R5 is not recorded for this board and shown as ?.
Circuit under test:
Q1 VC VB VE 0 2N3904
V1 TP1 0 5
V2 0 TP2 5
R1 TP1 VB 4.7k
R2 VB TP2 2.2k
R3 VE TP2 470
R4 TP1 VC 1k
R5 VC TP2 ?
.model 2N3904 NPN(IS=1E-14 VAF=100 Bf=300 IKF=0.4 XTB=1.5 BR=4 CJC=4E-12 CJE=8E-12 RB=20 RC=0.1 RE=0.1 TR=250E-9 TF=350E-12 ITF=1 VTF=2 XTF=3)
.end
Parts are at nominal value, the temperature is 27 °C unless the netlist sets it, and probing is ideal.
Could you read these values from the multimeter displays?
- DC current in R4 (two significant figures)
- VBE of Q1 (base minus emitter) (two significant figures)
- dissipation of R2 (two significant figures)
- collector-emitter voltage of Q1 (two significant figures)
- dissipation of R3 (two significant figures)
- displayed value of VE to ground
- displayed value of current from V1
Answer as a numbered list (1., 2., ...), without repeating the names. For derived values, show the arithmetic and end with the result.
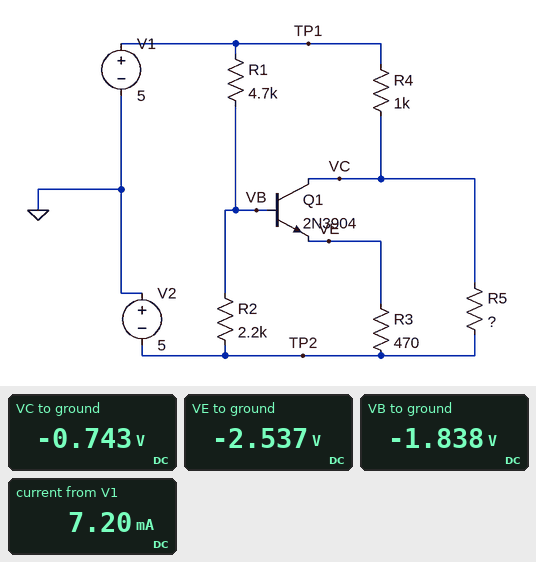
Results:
1. (5 V - (-743 mV)) / 1 kΩ = 5.7 mA
2. -1.838 V - (-2.537 V) = 700 mV
3. (-1.838 V - (-5 V))^2 / 2.2 kΩ = 4.5 mW
4. -743 mV - (-2.537 V) = 1.8 V
5. (-2.537 V - (-5 V))^2 / 470 Ω = 13 mW
6. -2.537 V
7. 7.20 mA
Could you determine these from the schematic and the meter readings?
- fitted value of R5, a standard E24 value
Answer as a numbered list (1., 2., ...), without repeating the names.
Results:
1. 8.2 kΩ
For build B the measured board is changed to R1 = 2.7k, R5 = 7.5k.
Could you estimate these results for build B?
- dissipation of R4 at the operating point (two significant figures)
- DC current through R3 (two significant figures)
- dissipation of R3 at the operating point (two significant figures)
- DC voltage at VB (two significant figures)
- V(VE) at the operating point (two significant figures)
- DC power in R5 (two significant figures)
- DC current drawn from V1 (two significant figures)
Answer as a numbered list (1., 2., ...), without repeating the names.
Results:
1. 46 mW
2. 6.8 mA
3. 22 mW
4. -1.1 V
5. -1.8 V
6. 1.4 mW
7. 9.0 mA
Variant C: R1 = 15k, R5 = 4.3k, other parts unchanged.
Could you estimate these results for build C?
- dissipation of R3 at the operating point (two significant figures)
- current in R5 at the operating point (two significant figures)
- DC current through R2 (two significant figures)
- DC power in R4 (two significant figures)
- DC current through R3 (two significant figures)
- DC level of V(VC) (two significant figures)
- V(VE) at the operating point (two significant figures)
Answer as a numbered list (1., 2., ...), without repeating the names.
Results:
1. 790 µW
2. 1.6 mA
3. 580 µA
4. 8.6 mW
5. 1.3 mA
6. 2.1 V
7. -4.4 V
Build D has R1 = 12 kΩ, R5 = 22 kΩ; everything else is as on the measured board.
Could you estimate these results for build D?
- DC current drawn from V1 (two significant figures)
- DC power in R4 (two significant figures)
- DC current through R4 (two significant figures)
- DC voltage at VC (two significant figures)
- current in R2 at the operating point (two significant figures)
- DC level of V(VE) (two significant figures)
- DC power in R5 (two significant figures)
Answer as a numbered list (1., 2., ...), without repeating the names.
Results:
1. 2.9 mA
2. 4.8 mW
3. 2.2 mA
4. 2.8 V
5. 700 µA
6. -4.1 V
7. 2.8 mW
